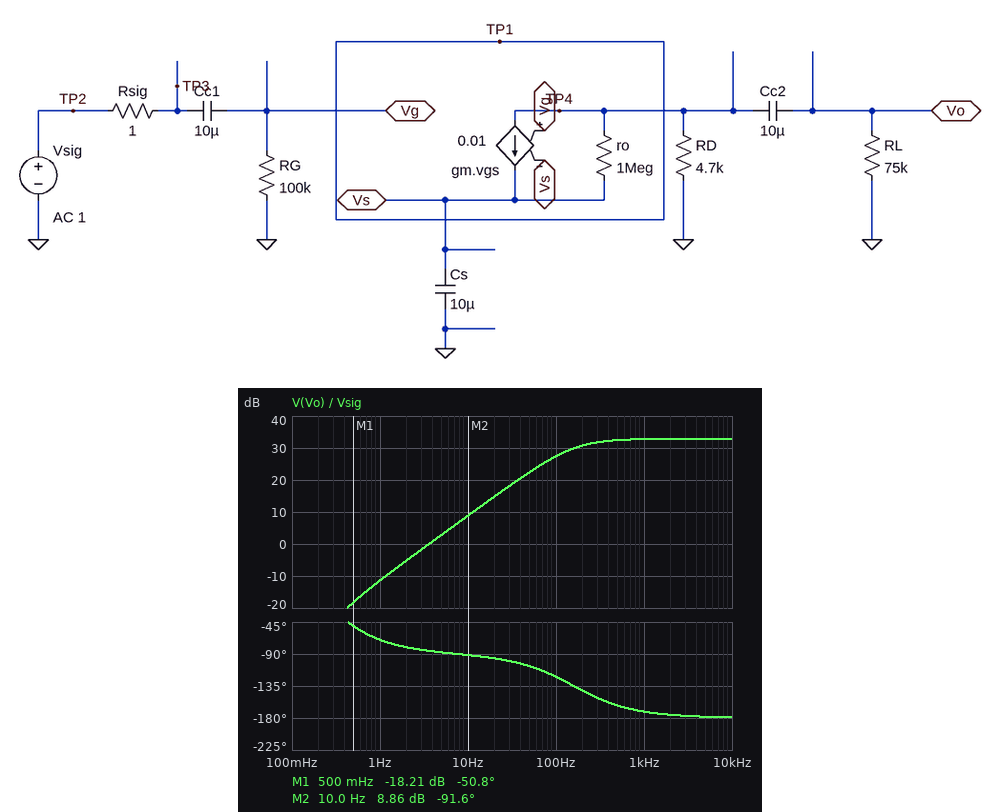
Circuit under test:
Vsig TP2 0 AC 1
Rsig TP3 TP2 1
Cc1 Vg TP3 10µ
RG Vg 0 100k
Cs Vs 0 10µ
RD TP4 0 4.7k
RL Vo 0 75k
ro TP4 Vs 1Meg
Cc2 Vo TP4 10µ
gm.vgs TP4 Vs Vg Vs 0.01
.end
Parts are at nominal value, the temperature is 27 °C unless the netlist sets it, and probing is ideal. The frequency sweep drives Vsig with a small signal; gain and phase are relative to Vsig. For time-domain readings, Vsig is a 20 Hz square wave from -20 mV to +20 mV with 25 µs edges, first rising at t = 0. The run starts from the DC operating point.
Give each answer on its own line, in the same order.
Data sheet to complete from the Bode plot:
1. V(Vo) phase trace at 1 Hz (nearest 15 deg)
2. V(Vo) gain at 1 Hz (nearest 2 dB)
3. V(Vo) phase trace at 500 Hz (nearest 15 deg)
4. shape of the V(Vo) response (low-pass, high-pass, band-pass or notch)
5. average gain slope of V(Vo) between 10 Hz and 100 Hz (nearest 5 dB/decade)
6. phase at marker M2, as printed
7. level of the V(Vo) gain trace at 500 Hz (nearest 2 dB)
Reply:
-75 deg
-12 dB
-165 deg
high-pass
20 dB/decade
-91.6 deg
32 dB
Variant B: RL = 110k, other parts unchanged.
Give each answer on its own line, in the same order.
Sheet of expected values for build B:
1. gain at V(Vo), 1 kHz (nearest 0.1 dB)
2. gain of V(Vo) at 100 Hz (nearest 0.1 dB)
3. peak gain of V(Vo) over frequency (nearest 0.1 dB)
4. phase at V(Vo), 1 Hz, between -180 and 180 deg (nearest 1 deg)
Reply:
32.9 dB
27.6 dB
33.0 dB
-73 deg
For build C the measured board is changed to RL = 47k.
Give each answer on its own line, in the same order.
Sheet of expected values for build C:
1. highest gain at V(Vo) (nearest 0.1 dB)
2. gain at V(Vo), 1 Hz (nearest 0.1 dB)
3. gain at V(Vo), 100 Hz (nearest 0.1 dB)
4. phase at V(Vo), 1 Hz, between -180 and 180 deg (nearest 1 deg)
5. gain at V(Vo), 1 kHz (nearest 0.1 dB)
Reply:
32.6 dB
-11.9 dB
27.1 dB
-64 deg
32.5 dB
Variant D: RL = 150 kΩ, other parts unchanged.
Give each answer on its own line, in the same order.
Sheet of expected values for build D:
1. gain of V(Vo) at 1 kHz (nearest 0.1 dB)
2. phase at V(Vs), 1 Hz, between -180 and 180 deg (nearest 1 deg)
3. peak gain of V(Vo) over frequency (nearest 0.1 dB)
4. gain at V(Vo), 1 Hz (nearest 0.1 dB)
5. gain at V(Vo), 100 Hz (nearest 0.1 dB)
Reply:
33.0 dB
9 deg
33.1 dB
-11.0 dB
27.7 dB
